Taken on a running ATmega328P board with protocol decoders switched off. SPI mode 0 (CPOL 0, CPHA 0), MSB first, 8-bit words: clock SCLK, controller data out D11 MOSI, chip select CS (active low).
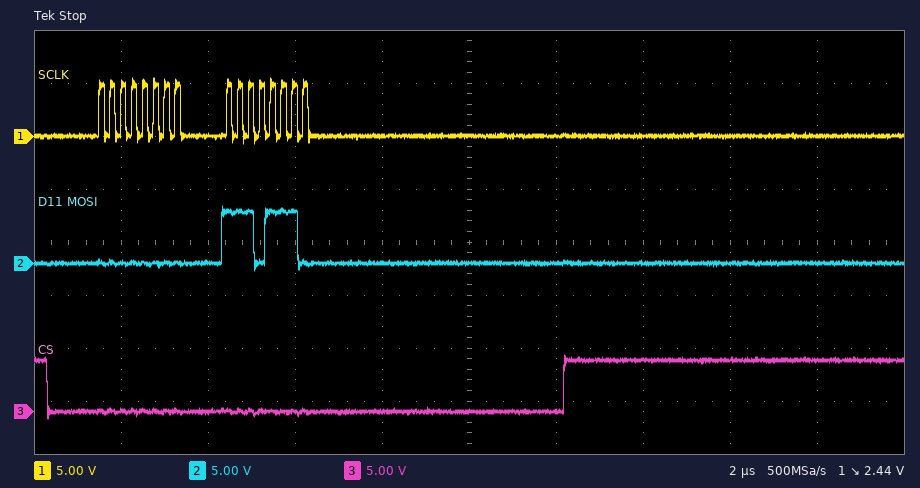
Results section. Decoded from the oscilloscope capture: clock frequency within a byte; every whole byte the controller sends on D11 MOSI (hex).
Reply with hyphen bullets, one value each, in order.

- 4 MHz
- 00 EE
